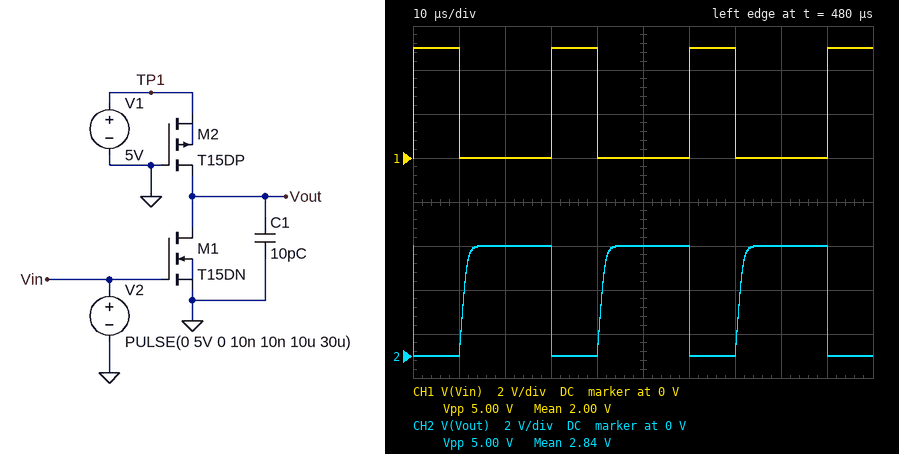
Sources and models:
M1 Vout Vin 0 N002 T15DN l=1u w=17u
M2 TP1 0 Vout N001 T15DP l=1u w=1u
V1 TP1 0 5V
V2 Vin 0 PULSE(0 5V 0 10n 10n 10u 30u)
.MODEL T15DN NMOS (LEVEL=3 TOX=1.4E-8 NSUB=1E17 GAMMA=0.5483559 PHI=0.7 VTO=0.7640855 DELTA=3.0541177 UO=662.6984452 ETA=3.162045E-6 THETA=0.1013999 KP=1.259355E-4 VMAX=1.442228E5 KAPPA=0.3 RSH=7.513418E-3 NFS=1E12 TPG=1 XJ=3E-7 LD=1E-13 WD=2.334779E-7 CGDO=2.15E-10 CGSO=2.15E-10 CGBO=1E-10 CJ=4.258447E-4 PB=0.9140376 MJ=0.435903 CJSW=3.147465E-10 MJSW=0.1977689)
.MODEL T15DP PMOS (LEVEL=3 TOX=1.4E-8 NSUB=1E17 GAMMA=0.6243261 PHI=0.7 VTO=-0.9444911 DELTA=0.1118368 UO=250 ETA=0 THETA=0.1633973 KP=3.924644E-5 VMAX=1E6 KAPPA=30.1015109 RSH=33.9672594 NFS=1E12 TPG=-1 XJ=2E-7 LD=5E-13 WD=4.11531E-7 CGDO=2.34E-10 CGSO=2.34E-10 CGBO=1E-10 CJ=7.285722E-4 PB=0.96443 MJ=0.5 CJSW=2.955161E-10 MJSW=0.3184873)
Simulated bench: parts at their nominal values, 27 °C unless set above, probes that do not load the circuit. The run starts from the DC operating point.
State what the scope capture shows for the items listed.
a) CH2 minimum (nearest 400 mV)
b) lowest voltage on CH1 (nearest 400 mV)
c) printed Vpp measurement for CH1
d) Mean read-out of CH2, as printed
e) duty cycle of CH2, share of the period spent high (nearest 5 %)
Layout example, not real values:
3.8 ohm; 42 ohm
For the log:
0 V; 0 V; 5.00 V; 2.84 V; 65 %
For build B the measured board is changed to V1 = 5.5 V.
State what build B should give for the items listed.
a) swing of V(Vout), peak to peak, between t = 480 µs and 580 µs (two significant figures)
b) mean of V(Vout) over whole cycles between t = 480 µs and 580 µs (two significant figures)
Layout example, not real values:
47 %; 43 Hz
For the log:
5.5 V; 3.5 V
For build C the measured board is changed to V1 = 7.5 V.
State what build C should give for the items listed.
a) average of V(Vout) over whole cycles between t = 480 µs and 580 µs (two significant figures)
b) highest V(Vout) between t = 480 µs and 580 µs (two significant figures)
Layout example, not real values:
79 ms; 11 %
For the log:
4.8 V; 7.5 V
